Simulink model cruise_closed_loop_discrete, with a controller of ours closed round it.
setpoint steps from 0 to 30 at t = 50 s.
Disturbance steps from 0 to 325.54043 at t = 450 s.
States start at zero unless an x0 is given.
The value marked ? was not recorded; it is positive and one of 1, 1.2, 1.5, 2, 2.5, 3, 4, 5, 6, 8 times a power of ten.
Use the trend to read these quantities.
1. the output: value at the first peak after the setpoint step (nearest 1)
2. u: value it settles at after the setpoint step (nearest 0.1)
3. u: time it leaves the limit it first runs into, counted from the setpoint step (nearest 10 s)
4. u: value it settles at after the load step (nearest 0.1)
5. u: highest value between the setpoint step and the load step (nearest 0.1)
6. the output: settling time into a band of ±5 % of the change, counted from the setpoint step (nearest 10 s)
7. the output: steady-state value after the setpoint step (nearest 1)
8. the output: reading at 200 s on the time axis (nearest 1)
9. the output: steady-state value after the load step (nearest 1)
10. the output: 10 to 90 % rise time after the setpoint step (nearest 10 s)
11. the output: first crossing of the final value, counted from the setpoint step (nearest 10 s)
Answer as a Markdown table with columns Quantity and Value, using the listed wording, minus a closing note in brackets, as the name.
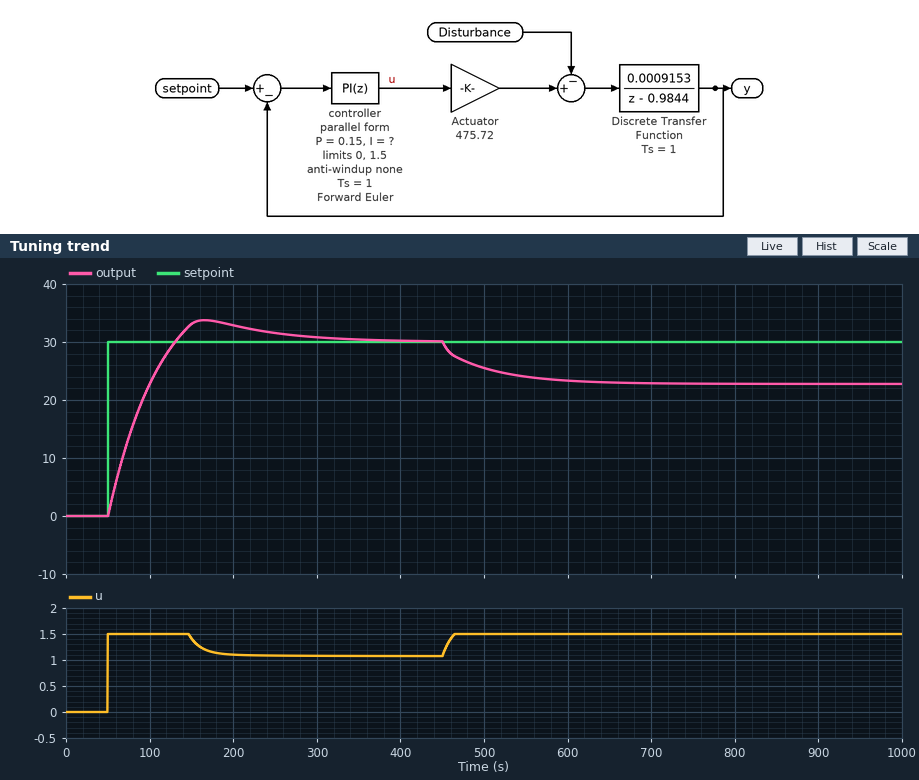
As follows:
| Quantity | Value |
|---|---|
| the output: value at the first peak after the setpoint step | 34 |
| u: value it settles at after the setpoint step | 1.1 |
| u: time it leaves the limit it first runs into, counted from the setpoint step | 100 s |
| u: value it settles at after the load step | 1.5 |
| u: highest value between the setpoint step and the load step | 1.5 |
| the output: settling time into a band of ±5 % of the change, counted from the setpoint step | 200 s |
| the output: steady-state value after the setpoint step | 30 |
| the output: reading at 200 s on the time axis | 33 |
| the output: steady-state value after the load step | 23 |
| the output: 10 to 90 % rise time after the setpoint step | 60 s |
| the output: first crossing of the final value, counted from the setpoint step | 80 s |
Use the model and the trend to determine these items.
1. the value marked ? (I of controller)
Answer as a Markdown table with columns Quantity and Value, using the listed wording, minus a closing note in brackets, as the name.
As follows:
| Quantity | Value |
|---|---|
| the value marked ? | 0.002 |
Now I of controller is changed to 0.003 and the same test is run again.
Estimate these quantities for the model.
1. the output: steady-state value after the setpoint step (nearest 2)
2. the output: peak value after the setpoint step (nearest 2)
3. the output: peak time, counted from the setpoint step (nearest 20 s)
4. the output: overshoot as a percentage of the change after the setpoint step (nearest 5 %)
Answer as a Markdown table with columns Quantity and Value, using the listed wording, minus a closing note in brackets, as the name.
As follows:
| Quantity | Value |
|---|---|
| the output: steady-state value after the setpoint step | 30 |
| the output: peak value after the setpoint step | 36 |
| the output: peak time, counted from the setpoint step | 140 s |
| the output: overshoot as a percentage of the change after the setpoint step | 20 % |
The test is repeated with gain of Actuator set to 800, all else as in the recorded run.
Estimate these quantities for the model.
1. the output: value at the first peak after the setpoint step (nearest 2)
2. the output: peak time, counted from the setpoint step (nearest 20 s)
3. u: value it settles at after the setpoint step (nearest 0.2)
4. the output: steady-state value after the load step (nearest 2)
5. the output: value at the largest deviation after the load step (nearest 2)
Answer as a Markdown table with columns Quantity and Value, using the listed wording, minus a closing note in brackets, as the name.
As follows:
| Quantity | Value |
|---|---|
| the output: value at the first peak after the setpoint step | 32 |
| the output: peak time, counted from the setpoint step | 60 s |
| u: value it settles at after the setpoint step | 0.6 |
| the output: steady-state value after the load step | 30 |
| the output: value at the largest deviation after the load step | 28 |
